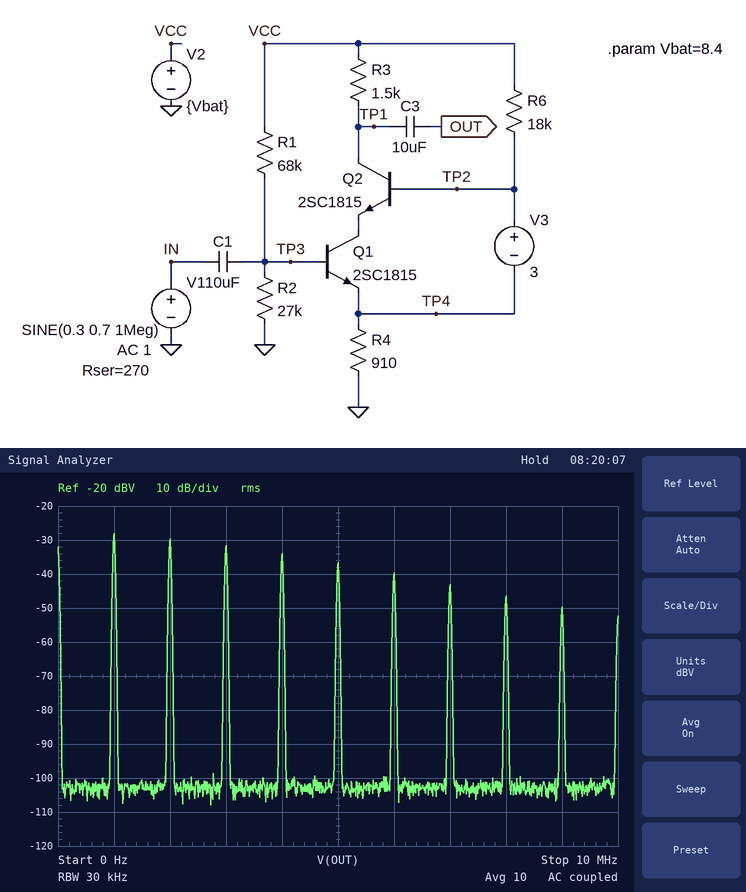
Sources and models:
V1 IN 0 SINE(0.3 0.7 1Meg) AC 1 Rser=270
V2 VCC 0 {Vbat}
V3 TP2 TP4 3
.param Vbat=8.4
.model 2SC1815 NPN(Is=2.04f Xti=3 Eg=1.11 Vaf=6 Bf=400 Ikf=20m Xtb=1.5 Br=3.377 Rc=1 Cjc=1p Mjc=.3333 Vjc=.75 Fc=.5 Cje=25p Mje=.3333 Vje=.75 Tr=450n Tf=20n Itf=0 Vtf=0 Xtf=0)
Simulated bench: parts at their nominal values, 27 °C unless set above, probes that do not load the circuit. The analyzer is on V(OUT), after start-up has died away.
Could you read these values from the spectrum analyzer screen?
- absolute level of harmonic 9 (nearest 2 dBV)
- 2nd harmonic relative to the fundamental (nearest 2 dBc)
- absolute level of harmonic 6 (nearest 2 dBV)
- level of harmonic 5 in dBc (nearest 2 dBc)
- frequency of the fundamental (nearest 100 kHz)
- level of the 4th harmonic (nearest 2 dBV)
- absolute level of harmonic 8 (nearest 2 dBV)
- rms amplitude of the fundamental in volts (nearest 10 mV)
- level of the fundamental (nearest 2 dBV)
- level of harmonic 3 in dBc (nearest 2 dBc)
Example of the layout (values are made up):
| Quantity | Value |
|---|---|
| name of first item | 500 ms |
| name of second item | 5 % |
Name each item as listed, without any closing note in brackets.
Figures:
| Quantity | Value |
|---|---|
| absolute level of harmonic 9 | -50 dBV |
| 2nd harmonic relative to the fundamental | -2 dBc |
| absolute level of harmonic 6 | -40 dBV |
| level of harmonic 5 in dBc | -8 dBc |
| frequency of the fundamental | 1.0 MHz |
| level of the 4th harmonic | -34 dBV |
| absolute level of harmonic 8 | -46 dBV |
| rms amplitude of the fundamental in volts | 40 mV |
| level of the fundamental | -28 dBV |
| level of harmonic 3 in dBc | -4 dBc |
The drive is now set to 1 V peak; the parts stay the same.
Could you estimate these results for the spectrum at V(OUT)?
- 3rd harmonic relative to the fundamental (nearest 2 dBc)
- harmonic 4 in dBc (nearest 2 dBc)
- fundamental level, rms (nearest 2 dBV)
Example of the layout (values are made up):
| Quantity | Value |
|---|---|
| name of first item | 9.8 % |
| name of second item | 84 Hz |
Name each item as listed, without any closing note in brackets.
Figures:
| Quantity | Value |
|---|---|
| 3rd harmonic relative to the fundamental | -6 dBc |
| harmonic 4 in dBc | -12 dBc |
| fundamental level, rms | -16 dBV |
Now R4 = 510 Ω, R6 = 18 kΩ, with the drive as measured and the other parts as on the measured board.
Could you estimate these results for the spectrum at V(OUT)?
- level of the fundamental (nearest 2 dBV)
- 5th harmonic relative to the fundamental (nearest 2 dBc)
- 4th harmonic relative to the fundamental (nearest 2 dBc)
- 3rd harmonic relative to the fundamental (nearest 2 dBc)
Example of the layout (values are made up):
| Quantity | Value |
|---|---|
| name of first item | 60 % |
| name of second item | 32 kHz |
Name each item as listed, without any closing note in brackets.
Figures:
| Quantity | Value |
|---|---|
| level of the fundamental | -16 dBV |
| 5th harmonic relative to the fundamental | -18 dBc |
| 4th harmonic relative to the fundamental | -10 dBc |
| 3rd harmonic relative to the fundamental | -6 dBc |
